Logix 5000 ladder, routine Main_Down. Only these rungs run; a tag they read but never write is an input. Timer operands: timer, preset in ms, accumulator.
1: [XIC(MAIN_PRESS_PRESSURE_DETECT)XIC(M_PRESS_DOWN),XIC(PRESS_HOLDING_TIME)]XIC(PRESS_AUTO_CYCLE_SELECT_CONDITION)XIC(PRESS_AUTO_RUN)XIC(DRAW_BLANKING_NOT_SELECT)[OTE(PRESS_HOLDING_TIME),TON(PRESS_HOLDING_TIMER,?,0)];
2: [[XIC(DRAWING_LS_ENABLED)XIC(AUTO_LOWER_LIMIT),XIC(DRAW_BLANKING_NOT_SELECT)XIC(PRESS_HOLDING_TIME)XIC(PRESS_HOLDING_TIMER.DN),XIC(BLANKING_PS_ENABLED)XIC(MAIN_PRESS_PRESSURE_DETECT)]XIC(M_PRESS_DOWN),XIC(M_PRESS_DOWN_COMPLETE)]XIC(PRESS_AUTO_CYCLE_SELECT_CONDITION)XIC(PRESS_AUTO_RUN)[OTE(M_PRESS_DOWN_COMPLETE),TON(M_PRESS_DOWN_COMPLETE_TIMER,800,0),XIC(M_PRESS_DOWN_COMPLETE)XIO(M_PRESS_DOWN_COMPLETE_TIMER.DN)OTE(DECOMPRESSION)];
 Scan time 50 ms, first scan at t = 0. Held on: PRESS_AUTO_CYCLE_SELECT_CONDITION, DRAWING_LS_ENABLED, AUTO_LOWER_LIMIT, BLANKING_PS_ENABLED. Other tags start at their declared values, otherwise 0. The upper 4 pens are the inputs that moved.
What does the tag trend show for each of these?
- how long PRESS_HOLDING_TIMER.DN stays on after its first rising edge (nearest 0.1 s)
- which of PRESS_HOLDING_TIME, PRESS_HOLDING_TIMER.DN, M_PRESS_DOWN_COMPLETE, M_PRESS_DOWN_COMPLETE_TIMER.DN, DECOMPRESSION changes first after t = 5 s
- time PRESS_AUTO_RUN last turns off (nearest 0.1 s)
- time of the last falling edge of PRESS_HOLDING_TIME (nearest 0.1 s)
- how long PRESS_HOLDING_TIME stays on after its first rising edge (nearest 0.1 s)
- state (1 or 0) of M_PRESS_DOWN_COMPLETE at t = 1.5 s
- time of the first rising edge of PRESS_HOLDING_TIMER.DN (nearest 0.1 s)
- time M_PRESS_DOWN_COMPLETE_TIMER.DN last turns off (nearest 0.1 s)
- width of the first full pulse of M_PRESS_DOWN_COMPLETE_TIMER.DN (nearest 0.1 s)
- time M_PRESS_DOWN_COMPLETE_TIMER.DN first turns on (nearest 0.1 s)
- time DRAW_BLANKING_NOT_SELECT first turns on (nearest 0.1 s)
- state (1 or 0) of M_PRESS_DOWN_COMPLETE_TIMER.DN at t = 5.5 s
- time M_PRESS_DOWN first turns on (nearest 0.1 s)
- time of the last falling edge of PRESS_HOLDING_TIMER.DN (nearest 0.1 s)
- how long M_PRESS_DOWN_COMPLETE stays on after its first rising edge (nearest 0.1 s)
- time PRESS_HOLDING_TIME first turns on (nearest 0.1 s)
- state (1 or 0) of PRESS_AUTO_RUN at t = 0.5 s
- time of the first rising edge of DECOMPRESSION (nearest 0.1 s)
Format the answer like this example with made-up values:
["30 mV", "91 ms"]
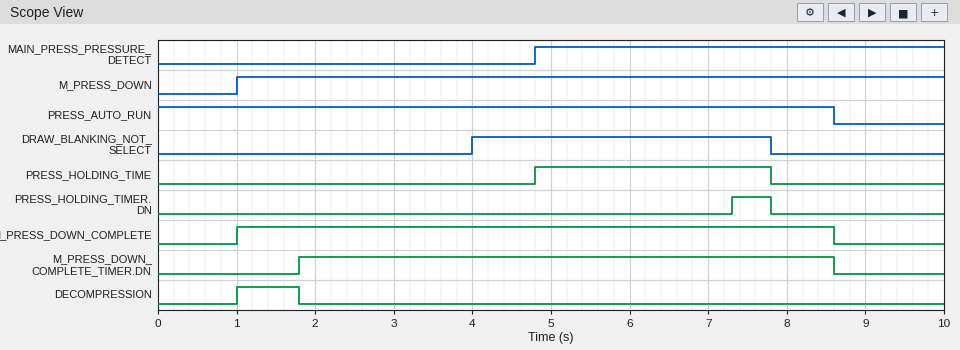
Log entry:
["0.5 s", "PRESS_HOLDING_TIMER.DN", "8.6 s", "7.8 s", "3.0 s", "1", "7.3 s", "8.6 s", "6.8 s", "1.8 s", "4.0 s", "1", "1.0 s", "7.8 s", "7.6 s", "4.8 s", "1", "1.0 s"]
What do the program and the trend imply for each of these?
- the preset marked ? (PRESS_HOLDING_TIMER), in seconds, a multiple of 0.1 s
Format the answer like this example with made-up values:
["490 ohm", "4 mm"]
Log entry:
["2.5 s"]
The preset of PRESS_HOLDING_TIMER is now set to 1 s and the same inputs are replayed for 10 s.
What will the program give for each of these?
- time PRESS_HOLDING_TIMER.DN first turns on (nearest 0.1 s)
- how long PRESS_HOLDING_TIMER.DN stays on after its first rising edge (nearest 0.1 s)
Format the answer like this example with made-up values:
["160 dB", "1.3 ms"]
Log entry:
["5.8 s", "2.0 s"]
